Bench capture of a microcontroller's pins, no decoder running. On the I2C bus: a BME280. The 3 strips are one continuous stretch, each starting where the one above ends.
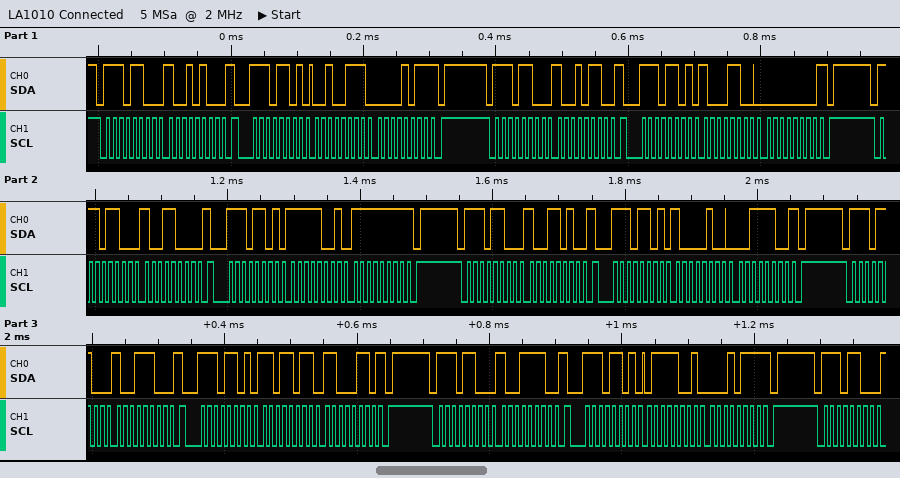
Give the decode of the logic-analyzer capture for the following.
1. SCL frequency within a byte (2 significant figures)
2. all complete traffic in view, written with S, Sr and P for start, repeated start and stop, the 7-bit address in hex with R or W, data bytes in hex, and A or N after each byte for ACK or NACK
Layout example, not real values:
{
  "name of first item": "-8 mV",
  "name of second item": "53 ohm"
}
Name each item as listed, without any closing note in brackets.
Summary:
{
  "SCL frequency within a byte": "100 kHz",
  "all complete traffic in view, written with S, Sr and P for start, repeated start and stop, the 7-bit address in hex with R or W, data bytes in hex, and A or N after each byte for ACK or NACK": "S 76W A 94 A Sr 76R A 27 A 0B N P S 76W A 96 A Sr 76R A 8C A 00 N P S 76W A 98 A Sr 76R A F9 A FF N P S 76W A 9A A Sr 76R A 84 A 3C N P S 76W A 9C A Sr 76R A DB A C6 N P S 76W A 9E A Sr 76R A 79 A 17 N P S 76W A"
}
